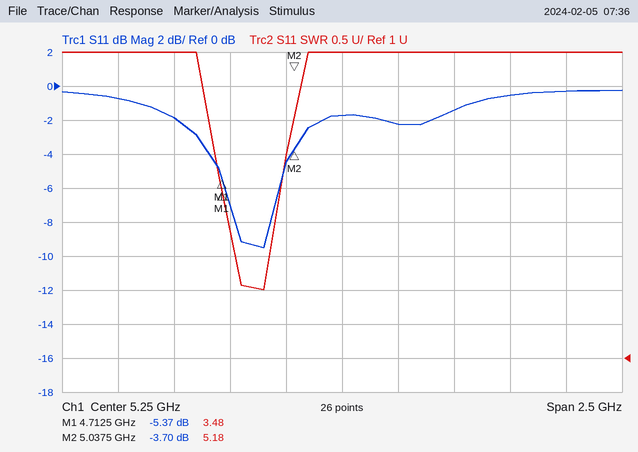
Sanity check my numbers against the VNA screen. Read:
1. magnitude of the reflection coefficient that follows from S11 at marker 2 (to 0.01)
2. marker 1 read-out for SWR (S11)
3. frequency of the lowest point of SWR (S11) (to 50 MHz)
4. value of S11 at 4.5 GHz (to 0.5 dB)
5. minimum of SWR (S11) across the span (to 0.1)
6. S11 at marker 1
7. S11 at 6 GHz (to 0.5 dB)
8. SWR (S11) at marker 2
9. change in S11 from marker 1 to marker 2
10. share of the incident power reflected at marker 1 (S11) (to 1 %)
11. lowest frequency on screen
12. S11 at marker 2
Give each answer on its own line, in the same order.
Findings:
0.65
3.48
4.90 GHz
-2.0 dB
2.0
-5.37 dB
-0.5 dB
5.18
1.67 dB
29 %
4 GHz
-3.70 dB
